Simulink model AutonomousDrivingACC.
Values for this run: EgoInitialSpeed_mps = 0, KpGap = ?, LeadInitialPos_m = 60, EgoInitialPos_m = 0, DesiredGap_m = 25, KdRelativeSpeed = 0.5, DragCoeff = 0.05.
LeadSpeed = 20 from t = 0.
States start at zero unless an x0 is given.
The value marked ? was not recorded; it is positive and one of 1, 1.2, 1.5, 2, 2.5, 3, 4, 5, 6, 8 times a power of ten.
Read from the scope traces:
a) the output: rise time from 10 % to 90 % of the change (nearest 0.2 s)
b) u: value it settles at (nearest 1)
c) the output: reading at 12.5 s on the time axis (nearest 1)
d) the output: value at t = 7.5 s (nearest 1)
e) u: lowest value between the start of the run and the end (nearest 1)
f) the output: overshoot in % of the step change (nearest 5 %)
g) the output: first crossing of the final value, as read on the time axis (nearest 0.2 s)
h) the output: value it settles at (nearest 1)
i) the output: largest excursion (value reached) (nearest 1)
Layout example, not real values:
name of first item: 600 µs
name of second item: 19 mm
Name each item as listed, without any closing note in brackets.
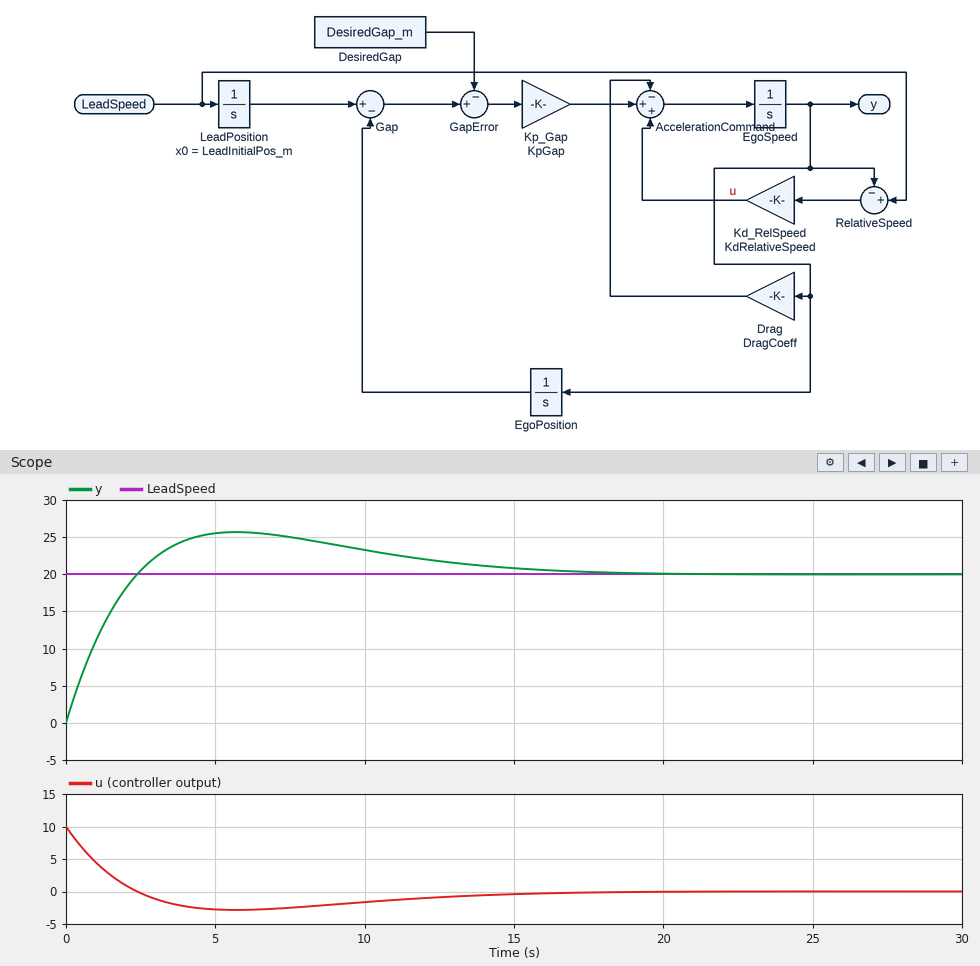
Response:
the output: rise time from 10 % to 90 % of the change: 1.8 s
u: value it settles at: 0
the output: reading at 12.5 s on the time axis: 22
the output: value at t = 7.5 s: 25
u: lowest value between the start of the run and the end: -3
the output: overshoot in % of the step change: 30 %
the output: first crossing of the final value, as read on the time axis: 2.4 s
the output: value it settles at: 20
the output: largest excursion (value reached): 26
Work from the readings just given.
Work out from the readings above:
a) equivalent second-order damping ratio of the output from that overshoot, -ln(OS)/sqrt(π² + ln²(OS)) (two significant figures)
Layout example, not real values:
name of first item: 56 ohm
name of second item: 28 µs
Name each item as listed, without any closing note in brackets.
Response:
equivalent second-order damping ratio of the output from that overshoot, -ln(OS)/sqrt(π² + ln²(OS)): 0.36
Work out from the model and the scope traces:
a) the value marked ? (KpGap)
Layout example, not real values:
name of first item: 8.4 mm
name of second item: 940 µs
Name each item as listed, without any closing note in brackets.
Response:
the value marked ?: 0.1
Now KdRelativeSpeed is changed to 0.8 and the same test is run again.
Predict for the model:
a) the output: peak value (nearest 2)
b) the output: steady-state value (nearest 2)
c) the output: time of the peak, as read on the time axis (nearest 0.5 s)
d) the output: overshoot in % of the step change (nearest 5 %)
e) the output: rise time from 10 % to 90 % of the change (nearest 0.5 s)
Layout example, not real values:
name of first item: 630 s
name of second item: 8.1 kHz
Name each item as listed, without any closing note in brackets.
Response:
the output: peak value: 24
the output: steady-state value: 20
the output: time of the peak, as read on the time axis: 5.0 s
the output: overshoot in % of the step change: 20 %
the output: rise time from 10 % to 90 % of the change: 1.5 s
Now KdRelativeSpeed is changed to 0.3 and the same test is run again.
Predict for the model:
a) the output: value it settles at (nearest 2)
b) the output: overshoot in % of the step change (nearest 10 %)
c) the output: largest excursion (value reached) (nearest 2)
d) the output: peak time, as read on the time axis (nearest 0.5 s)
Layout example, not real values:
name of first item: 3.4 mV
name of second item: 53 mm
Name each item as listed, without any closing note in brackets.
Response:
the output: value it settles at: 20
the output: overshoot in % of the step change: 40 %
the output: largest excursion (value reached): 28
the output: peak time, as read on the time axis: 6.5 s
